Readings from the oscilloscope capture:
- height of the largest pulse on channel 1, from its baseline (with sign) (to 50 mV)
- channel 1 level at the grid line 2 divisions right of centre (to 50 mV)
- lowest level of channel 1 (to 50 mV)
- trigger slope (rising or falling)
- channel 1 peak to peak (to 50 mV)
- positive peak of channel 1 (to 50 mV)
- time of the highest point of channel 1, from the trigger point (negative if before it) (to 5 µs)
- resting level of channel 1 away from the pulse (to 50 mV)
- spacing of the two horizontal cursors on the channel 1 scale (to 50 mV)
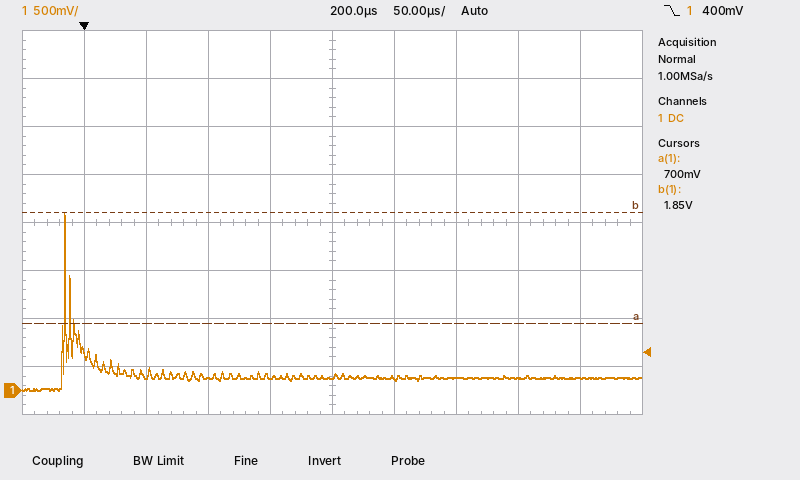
+1.70 V
150 mV
0 mV
falling
1.85 V
1.85 V
-15 µs
150 mV
1.15 V
